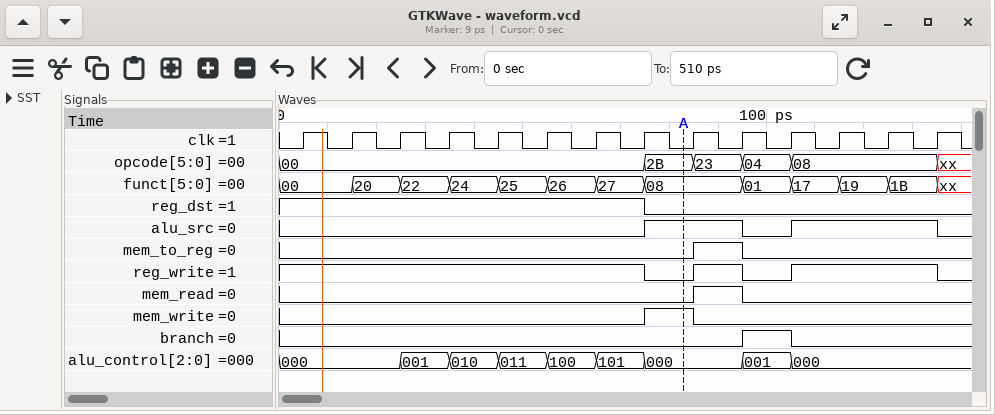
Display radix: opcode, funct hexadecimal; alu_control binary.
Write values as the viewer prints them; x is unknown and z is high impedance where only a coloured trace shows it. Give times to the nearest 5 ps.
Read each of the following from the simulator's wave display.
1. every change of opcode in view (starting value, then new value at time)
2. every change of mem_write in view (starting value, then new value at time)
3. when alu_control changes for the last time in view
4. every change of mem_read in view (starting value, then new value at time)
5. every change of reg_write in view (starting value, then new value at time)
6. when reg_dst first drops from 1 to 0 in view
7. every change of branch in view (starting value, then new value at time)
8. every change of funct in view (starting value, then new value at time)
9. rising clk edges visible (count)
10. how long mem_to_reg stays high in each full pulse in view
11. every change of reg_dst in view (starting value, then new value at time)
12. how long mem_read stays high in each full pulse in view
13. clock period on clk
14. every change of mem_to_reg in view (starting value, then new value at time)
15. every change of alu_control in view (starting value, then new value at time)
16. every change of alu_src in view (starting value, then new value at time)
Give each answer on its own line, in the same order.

00, 2B at 75 ps, 23 at 85 ps, 04 at 95 ps, 08 at 105 ps, xx at 135 ps
0, 1 at 75 ps, 0 at 85 ps
105 ps
0, 1 at 85 ps, 0 at 95 ps
1, 0 at 75 ps, 1 at 85 ps, 0 at 95 ps, 1 at 105 ps, 0 at 135 ps
75 ps
0, 1 at 95 ps, 0 at 105 ps
00, 20 at 15 ps, 22 at 25 ps, 24 at 35 ps, 25 at 45 ps, 26 at 55 ps, 27 at 65 ps, 08 at 75 ps, 01 at 95 ps, 17 at 105 ps, 19 at 115 ps, 1B at 125 ps, xx at 135 ps
14
10 ps
1, 0 at 75 ps
10 ps
10 ps
0, 1 at 85 ps, 0 at 95 ps
000, 001 at 25 ps, 010 at 35 ps, 011 at 45 ps, 100 at 55 ps, 101 at 65 ps, 000 at 75 ps, 001 at 95 ps, 000 at 105 ps
0, 1 at 75 ps, 0 at 95 ps, 1 at 105 ps, 0 at 135 ps
